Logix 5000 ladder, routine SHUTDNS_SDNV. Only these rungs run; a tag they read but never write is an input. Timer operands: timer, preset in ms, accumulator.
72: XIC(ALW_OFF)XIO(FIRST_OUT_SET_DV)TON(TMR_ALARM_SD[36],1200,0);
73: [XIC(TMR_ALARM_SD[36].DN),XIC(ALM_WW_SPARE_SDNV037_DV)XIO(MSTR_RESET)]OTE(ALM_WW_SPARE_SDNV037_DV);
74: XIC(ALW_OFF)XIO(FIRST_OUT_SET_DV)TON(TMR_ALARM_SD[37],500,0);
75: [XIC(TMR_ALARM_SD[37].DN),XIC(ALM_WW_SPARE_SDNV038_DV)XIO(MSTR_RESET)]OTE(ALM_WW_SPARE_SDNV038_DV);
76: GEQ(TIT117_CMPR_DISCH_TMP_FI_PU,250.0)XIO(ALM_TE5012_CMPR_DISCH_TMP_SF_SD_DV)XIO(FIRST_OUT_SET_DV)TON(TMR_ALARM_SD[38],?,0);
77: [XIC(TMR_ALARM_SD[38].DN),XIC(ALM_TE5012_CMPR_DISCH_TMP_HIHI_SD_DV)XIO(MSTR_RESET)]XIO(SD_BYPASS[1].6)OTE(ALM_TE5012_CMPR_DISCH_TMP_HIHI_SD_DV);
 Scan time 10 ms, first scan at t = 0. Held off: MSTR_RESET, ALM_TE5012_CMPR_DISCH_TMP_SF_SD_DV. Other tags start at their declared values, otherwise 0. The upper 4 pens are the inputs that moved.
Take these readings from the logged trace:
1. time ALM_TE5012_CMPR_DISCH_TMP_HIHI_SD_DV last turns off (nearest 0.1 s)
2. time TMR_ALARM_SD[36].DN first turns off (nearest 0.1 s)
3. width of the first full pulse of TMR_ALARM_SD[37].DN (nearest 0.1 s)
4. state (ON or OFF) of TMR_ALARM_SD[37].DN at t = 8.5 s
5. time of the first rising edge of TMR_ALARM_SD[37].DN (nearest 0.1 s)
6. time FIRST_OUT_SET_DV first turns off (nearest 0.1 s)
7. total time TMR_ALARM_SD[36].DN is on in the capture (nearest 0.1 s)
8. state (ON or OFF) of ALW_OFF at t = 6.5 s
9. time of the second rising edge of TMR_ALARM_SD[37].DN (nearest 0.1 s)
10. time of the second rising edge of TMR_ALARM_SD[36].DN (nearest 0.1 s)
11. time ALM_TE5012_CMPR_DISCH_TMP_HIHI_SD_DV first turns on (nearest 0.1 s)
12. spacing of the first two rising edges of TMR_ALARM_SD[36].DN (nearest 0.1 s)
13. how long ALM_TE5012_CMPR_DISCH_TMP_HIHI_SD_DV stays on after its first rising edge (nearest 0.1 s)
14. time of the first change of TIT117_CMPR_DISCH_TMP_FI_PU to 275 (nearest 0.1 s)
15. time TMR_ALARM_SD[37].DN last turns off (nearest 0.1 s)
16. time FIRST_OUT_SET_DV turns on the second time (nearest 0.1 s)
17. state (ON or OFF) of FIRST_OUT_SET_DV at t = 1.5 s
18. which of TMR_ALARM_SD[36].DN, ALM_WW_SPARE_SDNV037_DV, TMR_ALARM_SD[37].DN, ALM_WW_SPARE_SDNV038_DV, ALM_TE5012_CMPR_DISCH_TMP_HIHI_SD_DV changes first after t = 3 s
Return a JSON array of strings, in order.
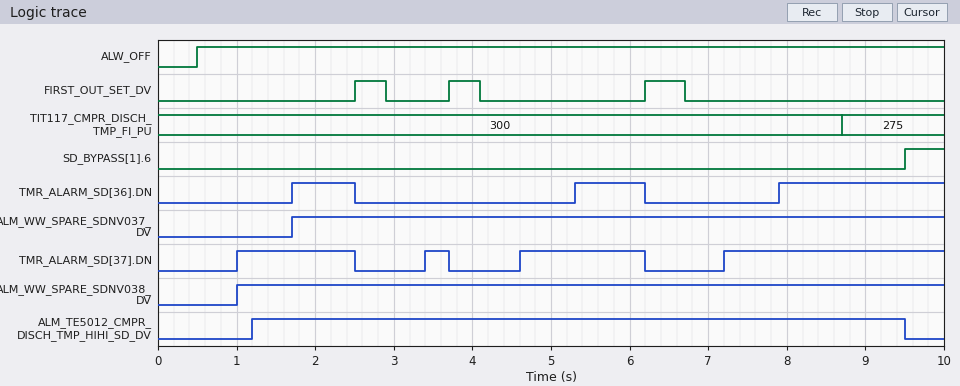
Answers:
["9.5 s", "2.5 s", "1.5 s", "ON", "1.0 s", "2.9 s", "3.8 s", "ON", "3.4 s", "5.3 s", "1.2 s", "3.6 s", "8.3 s", "8.7 s", "6.2 s", "3.7 s", "OFF", "TMR_ALARM_SD[37].DN"]
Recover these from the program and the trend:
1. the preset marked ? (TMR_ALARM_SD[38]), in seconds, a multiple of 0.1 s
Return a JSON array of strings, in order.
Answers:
["1.2 s"]
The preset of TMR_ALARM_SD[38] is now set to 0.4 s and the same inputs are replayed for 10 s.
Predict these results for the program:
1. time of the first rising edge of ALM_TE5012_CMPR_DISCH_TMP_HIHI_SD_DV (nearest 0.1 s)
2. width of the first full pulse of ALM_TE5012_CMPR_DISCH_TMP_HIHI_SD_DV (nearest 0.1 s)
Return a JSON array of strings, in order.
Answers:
["0.4 s", "9.1 s"]
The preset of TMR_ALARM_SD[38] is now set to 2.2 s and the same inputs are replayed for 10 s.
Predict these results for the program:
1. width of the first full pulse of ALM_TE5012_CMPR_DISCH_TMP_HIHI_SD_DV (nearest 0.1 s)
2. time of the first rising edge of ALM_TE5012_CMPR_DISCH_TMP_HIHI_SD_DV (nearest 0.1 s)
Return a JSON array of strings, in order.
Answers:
["7.3 s", "2.2 s"]
